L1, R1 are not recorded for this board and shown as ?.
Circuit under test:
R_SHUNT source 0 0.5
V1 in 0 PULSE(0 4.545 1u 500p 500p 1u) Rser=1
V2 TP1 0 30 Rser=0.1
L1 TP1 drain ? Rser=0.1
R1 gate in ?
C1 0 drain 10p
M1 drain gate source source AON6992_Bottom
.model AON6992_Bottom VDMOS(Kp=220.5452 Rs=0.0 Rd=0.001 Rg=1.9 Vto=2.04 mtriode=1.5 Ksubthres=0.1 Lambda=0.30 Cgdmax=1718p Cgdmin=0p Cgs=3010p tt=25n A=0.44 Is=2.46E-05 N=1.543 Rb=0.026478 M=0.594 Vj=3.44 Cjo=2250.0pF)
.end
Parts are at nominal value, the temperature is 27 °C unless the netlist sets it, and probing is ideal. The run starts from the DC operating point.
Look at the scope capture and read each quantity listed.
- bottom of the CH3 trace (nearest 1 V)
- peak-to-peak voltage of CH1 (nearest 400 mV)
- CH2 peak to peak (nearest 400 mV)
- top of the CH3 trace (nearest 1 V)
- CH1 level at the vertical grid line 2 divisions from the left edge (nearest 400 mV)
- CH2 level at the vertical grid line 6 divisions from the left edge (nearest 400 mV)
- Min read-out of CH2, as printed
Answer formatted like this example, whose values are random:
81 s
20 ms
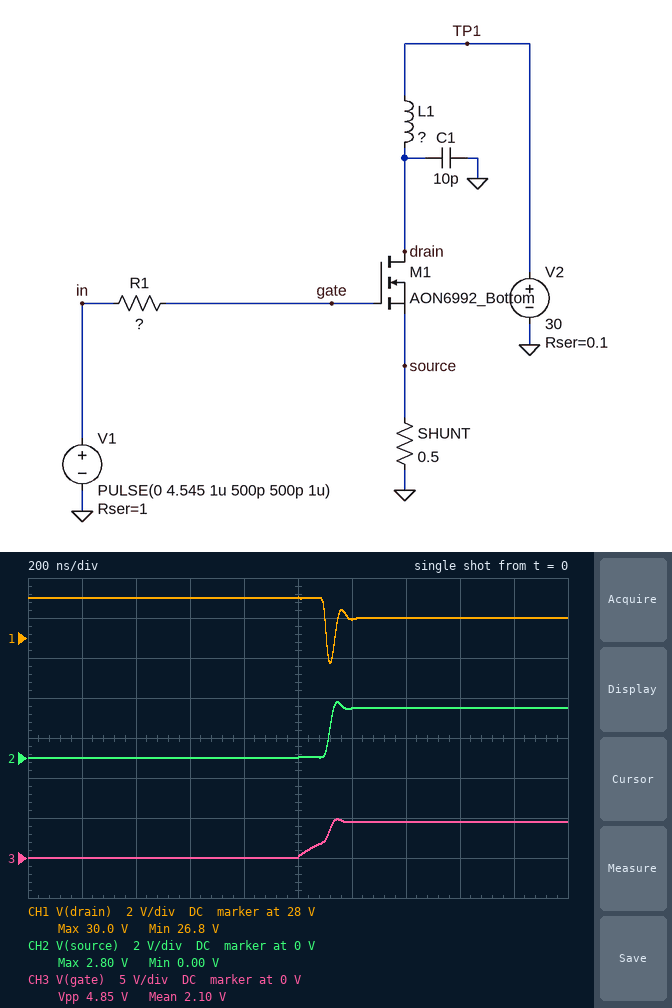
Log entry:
0 V
3.2 V
2.8 V
5 V
30.0 V
2.4 V
0.00 V
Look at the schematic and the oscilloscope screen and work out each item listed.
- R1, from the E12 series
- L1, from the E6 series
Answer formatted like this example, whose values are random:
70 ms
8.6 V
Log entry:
56 Ω
15 nH
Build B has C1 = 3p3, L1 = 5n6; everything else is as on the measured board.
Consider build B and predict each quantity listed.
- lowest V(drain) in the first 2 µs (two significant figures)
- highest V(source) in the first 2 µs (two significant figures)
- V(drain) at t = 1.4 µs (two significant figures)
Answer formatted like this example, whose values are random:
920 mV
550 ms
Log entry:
28 V
2.5 V
29 V
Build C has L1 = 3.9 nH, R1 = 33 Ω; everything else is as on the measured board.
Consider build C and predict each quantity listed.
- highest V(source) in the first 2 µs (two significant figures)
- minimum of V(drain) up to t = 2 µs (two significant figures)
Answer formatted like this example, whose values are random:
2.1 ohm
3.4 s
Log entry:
2.5 V
28 V
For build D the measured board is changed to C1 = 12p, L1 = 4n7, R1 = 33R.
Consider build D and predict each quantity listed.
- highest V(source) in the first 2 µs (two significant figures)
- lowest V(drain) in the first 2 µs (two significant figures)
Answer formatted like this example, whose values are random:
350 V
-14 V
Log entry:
2.6 V
28 V
